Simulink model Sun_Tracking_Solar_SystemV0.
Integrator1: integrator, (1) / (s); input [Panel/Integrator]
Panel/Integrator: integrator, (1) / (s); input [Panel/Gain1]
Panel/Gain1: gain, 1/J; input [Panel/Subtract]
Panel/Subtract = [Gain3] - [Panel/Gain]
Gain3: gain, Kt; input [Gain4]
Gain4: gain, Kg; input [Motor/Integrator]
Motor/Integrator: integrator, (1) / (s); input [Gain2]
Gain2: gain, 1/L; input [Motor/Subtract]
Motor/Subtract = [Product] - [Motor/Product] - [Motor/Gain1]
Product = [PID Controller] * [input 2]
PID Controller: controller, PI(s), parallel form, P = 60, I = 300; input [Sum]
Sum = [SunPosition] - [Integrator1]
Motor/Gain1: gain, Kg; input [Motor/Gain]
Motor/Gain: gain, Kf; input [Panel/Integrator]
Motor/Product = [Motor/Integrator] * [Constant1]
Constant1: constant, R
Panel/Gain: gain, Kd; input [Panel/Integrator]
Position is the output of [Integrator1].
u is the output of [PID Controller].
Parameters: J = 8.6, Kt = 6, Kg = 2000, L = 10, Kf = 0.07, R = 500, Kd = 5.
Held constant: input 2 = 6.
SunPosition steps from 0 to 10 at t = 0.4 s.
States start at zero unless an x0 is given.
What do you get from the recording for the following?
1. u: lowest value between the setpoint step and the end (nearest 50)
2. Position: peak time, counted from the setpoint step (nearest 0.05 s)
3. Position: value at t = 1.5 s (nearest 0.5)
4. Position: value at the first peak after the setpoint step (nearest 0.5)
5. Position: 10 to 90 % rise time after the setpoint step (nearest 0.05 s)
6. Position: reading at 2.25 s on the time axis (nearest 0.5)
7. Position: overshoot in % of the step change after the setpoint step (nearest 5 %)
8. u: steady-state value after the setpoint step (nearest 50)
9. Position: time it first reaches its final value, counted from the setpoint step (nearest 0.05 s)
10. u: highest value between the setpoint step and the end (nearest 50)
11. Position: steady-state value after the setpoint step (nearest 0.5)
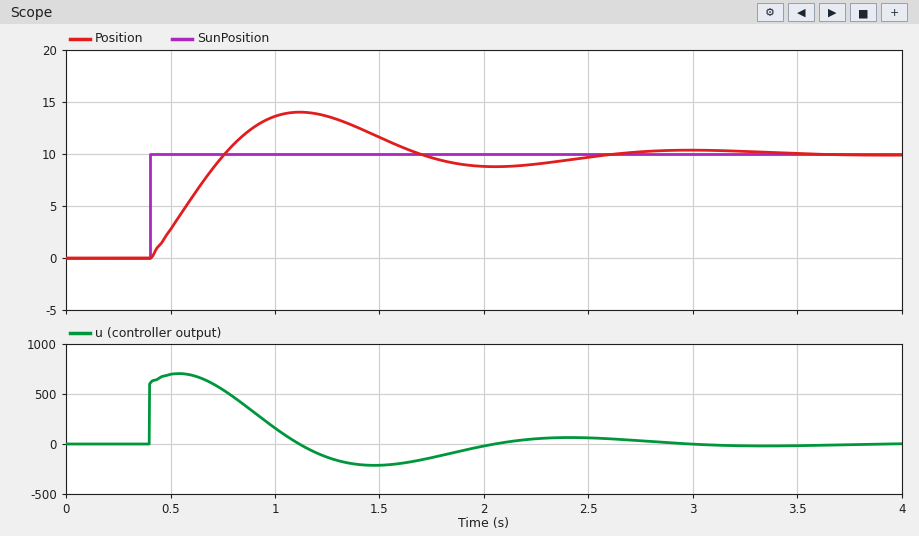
-200
0.70 s
11.5
14.0
0.30 s
9.0
40 %
0
0.35 s
700
10.0
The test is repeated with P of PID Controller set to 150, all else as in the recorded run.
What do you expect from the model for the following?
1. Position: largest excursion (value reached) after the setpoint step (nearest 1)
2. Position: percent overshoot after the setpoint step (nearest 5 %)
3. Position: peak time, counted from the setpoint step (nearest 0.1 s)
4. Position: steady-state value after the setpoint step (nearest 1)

12
15 %
0.6 s
10
